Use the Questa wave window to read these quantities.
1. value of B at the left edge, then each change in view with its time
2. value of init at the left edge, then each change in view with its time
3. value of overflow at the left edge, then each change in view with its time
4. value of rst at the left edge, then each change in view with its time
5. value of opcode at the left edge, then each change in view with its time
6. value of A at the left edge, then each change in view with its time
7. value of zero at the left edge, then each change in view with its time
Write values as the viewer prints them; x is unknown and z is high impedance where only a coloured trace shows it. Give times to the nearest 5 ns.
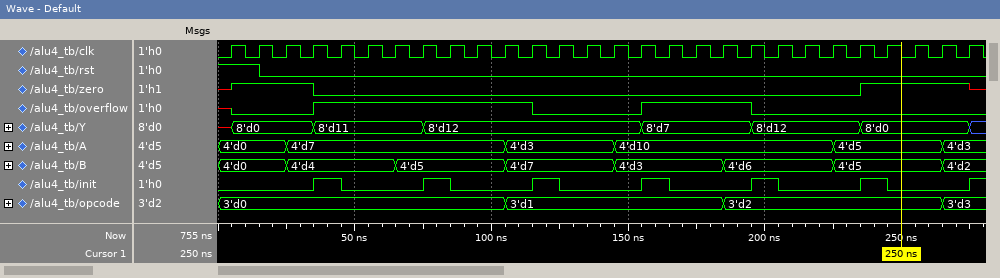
4'd0, 4'd4 at 25 ns, 4'd5 at 65 ns, 4'd7 at 105 ns, 4'd3 at 145 ns, 4'd6 at 185 ns, 4'd5 at 225 ns, 4'd2 at 265 ns
0, 1 at 35 ns, 0 at 45 ns, 1 at 75 ns, 0 at 85 ns, 1 at 115 ns, 0 at 125 ns, 1 at 155 ns, 0 at 165 ns, 1 at 195 ns, 0 at 205 ns, 1 at 235 ns, 0 at 245 ns, 1 at 275 ns
x, 0 at 5 ns, 1 at 35 ns, 0 at 115 ns, 1 at 155 ns, 0 at 195 ns
1, 0 at 15 ns
3'd0, 3'd1 at 105 ns, 3'd2 at 185 ns, 3'd3 at 265 ns
4'd0, 4'd7 at 25 ns, 4'd3 at 105 ns, 4'd10 at 145 ns, 4'd5 at 225 ns, 4'd3 at 265 ns
x, 1 at 5 ns, 0 at 35 ns, 1 at 235 ns, x at 275 ns
